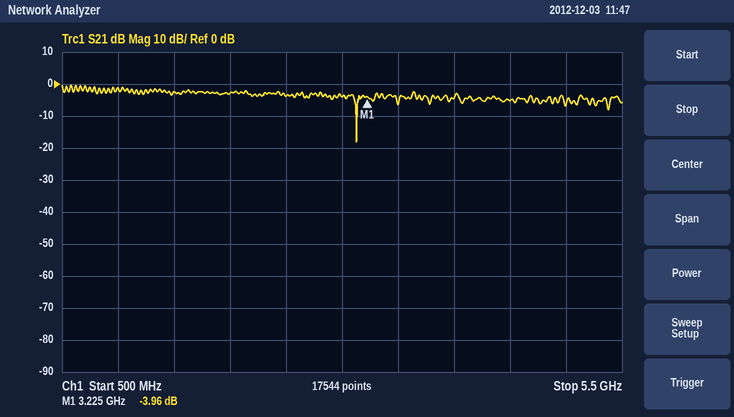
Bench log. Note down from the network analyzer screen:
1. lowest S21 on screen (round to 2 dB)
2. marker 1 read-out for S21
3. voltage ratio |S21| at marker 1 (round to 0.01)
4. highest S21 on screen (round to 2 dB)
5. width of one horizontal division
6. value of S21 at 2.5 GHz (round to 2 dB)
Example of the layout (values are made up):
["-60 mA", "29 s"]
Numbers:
["-18 dB", "-3.96 dB", "0.63", "0 dB", "500 MHz", "-4 dB"]
